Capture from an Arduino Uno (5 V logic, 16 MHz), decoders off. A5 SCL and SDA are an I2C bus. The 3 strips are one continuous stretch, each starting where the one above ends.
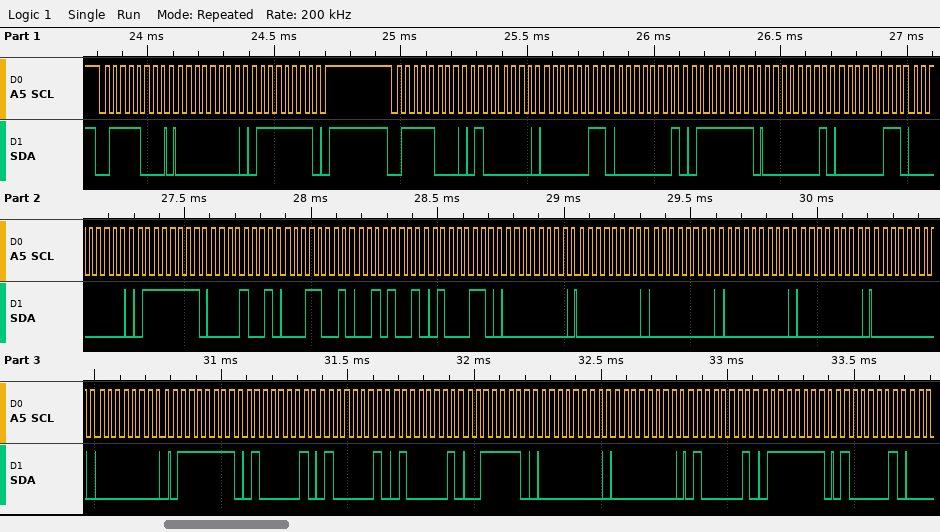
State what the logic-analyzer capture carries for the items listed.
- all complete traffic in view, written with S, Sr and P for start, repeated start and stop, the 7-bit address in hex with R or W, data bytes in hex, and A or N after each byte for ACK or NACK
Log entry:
S 3CW A 00 A 7F A P S 3CW A 40 A 03 A 01 A 7F A 01 A 03 A 00 A 7F A 09 A 19 A 29 A 46 A 00 A 00 A 00 A 00 A 00 A 00 A 00 A 7F A 41 A 41 A 41 A 3E A 00 A 00 A 41 A 7F A 41 A
